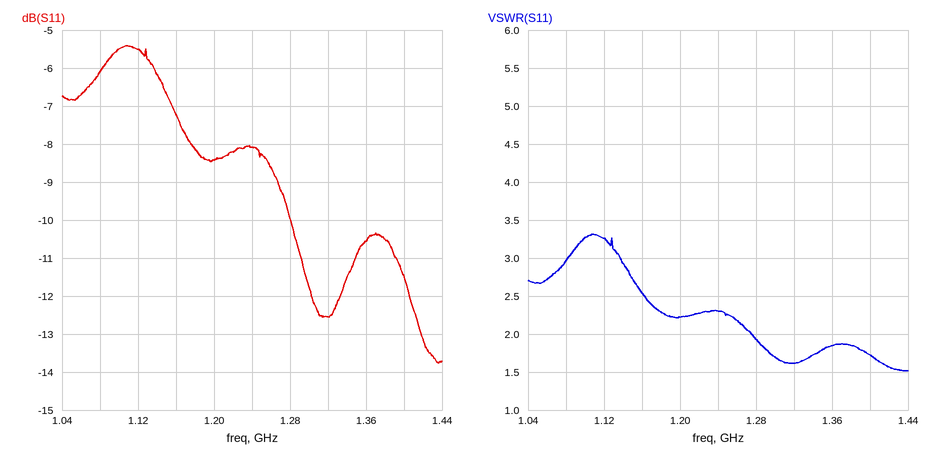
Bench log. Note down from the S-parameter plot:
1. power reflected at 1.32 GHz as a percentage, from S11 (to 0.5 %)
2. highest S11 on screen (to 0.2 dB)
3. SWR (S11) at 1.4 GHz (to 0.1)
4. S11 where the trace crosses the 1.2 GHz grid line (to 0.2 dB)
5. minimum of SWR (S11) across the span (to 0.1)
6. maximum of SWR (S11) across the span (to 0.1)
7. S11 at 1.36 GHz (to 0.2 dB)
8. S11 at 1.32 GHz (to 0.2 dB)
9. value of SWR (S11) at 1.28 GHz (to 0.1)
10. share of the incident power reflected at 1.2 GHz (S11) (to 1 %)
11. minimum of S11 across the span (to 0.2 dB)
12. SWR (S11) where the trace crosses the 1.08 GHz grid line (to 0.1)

5.5 %
-5.4 dB
1.7
-8.4 dB
1.5
3.3
-10.6 dB
-12.6 dB
1.9
14 %
-13.8 dB
3.0
